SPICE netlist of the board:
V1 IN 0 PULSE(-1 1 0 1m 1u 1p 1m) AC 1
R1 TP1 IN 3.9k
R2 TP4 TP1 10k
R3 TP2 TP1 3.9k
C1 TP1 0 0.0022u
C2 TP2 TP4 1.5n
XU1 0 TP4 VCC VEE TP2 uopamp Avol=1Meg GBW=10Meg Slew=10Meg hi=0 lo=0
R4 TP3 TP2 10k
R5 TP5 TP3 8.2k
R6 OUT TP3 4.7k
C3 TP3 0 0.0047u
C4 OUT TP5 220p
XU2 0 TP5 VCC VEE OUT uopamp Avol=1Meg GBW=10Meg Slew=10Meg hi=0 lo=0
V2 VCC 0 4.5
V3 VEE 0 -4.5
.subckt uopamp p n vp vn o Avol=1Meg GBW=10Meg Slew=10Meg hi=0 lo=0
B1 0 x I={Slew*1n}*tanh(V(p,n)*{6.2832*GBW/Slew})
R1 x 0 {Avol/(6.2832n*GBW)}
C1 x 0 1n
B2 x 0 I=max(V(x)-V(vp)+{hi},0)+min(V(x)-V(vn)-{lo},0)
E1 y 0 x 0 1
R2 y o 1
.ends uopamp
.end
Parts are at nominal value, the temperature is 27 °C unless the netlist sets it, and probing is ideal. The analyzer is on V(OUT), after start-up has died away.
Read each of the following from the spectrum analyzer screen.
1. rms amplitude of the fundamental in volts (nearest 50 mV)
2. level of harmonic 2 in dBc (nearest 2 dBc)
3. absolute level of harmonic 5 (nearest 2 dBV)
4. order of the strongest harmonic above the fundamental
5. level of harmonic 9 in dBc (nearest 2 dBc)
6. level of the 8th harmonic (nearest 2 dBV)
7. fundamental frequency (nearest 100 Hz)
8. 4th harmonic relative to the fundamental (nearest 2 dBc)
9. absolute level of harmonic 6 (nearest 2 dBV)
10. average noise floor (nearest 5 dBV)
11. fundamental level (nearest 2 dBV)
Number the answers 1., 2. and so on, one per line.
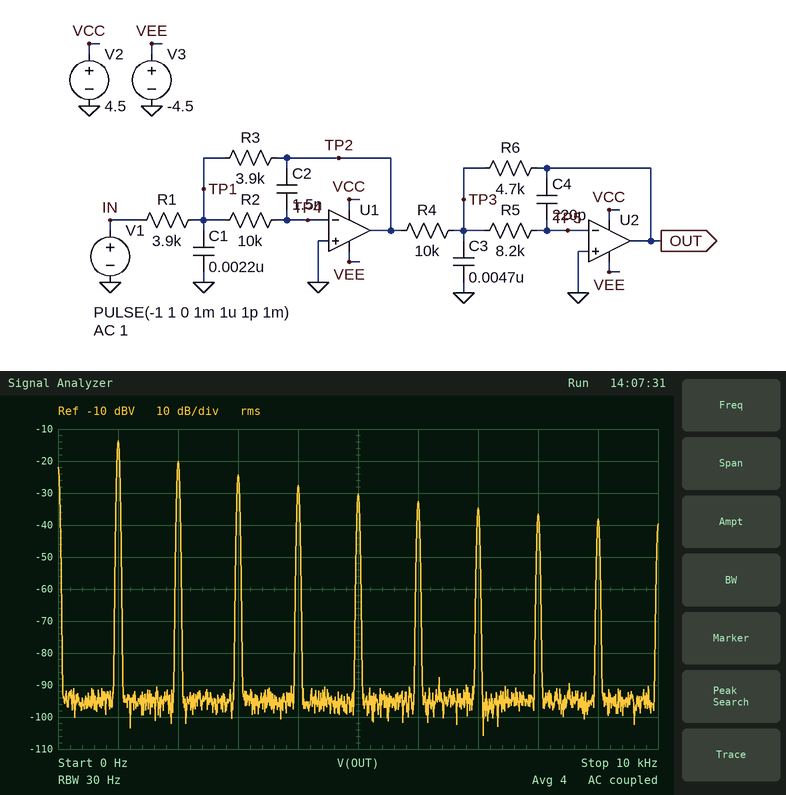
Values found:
1. 200 mV
2. -6 dBc
3. -30 dBV
4. 2
5. -24 dBc
6. -36 dBV
7. 1.0 kHz
8. -14 dBc
9. -32 dBV
10. -95 dBV
11. -14 dBV
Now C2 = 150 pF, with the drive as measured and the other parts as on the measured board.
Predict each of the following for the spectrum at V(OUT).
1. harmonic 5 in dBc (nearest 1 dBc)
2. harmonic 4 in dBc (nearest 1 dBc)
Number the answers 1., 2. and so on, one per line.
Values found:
1. -14 dBc
2. -12 dBc
